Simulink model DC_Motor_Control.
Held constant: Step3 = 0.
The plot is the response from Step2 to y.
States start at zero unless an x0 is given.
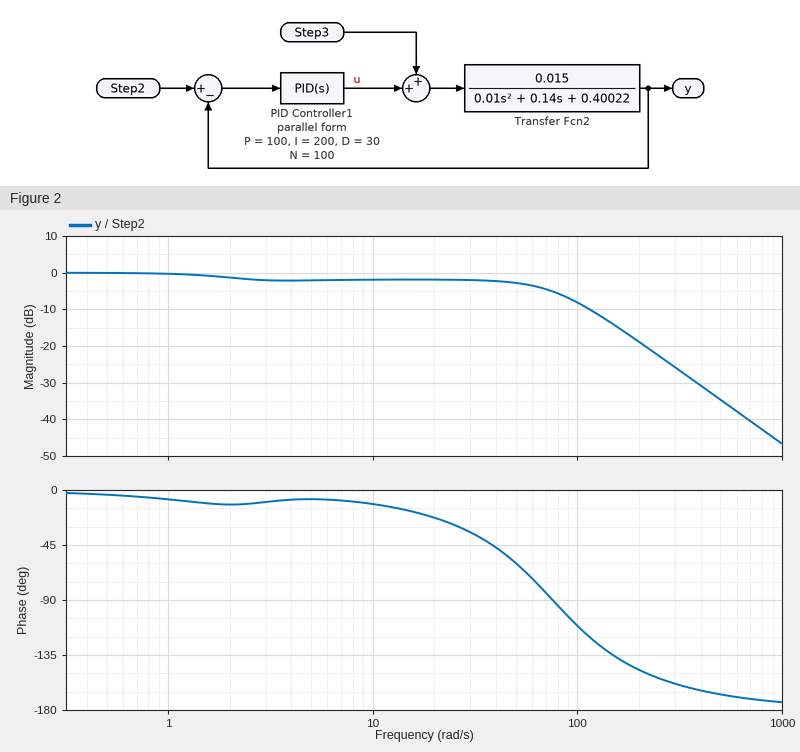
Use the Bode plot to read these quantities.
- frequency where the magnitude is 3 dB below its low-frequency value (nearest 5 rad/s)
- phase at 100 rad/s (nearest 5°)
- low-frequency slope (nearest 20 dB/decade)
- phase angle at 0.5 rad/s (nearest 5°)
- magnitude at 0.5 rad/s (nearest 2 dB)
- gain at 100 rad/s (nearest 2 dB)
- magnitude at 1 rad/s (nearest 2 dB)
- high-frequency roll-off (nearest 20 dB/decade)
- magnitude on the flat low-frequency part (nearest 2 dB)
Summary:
55 rad/s
-110°
0 dB/decade
-5°
0 dB
-8 dB
0 dB
-40 dB/decade
0 dB
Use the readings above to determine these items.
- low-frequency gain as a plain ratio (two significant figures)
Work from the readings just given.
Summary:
1.0
